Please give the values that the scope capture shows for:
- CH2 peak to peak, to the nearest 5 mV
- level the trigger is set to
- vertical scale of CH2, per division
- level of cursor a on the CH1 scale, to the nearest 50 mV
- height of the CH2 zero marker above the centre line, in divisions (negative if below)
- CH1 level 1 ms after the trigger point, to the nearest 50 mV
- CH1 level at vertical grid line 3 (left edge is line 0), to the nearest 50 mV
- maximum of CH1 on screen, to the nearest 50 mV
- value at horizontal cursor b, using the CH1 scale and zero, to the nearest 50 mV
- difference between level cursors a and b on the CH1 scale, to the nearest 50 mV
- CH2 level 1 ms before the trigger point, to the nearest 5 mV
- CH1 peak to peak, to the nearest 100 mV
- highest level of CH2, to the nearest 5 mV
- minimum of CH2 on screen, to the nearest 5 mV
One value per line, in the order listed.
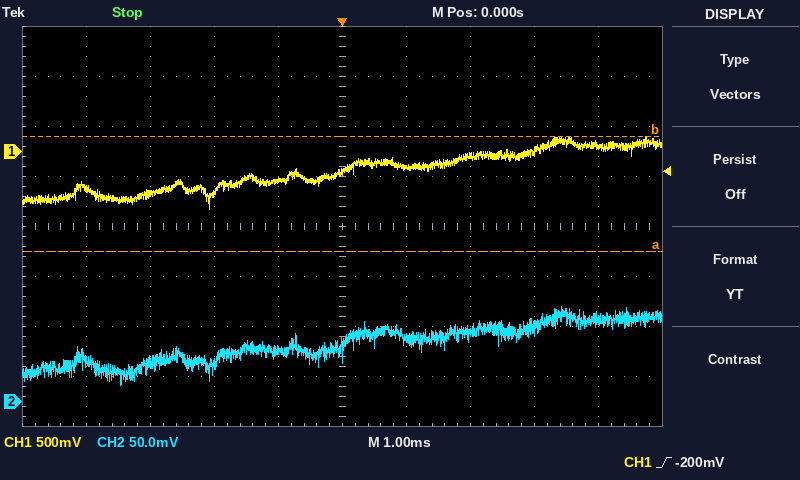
80 mV
-200 mV
50 mV
-1.00 V
-3.5 div
-150 mV
-400 mV
150 mV
150 mV
1.15 V
50 mV
700 mV
95 mV
15 mV
